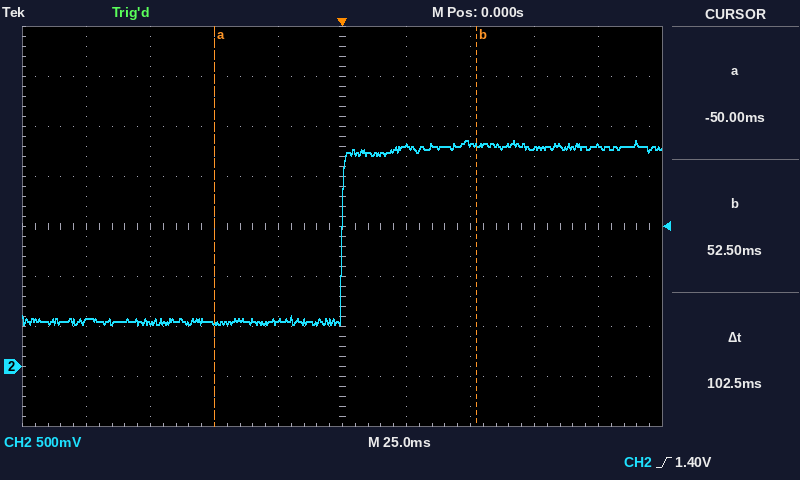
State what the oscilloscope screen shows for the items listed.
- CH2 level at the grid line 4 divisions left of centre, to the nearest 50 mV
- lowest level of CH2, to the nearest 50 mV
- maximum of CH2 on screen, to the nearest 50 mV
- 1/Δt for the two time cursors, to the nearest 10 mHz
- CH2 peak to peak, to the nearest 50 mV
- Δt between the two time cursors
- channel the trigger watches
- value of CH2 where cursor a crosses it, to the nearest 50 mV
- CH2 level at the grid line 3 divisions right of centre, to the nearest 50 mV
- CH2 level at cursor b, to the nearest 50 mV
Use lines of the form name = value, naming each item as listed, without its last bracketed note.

CH2 level at the grid line 4 divisions left of centre, to the nearest 50 mV = 450 mV
lowest level of CH2, to the nearest 50 mV = 400 mV
maximum of CH2 on screen, to the nearest 50 mV = 2.25 V
1/Δt for the two time cursors, to the nearest 10 mHz = 9.76 Hz
CH2 peak to peak, to the nearest 50 mV = 1.85 V
Δt between the two time cursors = 102.5 ms
channel the trigger watches = CH2
value of CH2 where cursor a crosses it, to the nearest 50 mV = 450 mV
CH2 level at the grid line 3 divisions right of centre, to the nearest 50 mV = 2.20 V
CH2 level at cursor b, to the nearest 50 mV = 2.20 V
